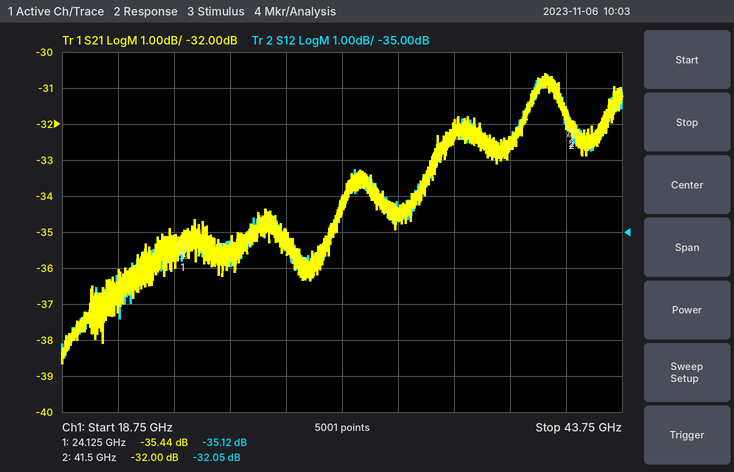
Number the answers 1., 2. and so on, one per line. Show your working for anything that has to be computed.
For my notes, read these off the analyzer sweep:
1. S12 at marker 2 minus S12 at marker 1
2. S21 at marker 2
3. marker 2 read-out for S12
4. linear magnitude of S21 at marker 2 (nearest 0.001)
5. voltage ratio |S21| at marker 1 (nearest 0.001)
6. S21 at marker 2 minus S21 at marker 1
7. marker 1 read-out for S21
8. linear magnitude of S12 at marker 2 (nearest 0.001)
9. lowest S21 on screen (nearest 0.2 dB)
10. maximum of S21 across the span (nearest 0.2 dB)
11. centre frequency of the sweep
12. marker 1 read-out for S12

1. -32.05 − (-35.12) = 3.07 dB
2. -32.00 dB
3. -32.05 dB
4. 10^(-32/20) ≈ 0.025
5. 10^(-35.44/20) ≈ 0.017
6. -32 − (-35.44) = 3.44 dB
7. -35.44 dB
8. 10^(-32.05/20) ≈ 0.025
9. -38.6 dB
10. -30.6 dB
11. 31.25 GHz
12. -35.12 dB
